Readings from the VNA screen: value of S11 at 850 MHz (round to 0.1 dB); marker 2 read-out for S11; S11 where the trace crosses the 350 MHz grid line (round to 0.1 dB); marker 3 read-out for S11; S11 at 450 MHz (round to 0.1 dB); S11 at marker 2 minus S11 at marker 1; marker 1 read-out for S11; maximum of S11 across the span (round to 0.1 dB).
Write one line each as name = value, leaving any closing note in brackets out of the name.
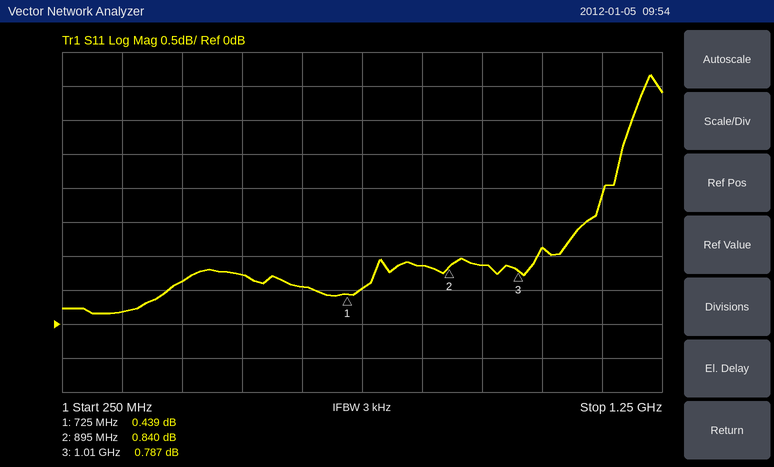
value of S11 at 850 MHz = 0.9 dB
marker 2 read-out for S11 = 0.840 dB
S11 where the trace crosses the 350 MHz grid line = 0.2 dB
marker 3 read-out for S11 = 0.787 dB
S11 at 450 MHz = 0.6 dB
S11 at marker 2 minus S11 at marker 1 = 0.401 dB
marker 1 read-out for S11 = 0.439 dB
maximum of S11 across the span = 3.7 dB
